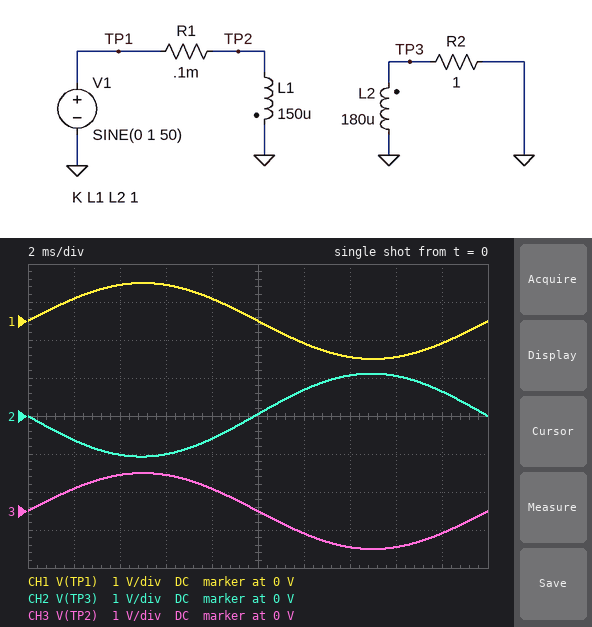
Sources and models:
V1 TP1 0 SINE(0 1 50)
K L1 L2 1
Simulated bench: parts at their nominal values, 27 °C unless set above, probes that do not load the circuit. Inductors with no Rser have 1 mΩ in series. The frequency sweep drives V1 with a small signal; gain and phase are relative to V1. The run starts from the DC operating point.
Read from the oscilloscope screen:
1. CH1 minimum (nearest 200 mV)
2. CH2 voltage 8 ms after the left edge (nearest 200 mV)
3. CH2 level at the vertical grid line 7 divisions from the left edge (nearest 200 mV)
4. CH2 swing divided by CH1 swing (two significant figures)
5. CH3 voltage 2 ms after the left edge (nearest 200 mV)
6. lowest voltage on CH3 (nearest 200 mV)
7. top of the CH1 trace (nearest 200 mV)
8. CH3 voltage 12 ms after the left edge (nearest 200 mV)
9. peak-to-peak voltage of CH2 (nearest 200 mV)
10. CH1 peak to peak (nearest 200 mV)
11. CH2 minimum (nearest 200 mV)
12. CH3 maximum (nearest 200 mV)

-1.0 V
-600 mV
1.0 V
1.1
600 mV
-1.0 V
1.0 V
-600 mV
2.2 V
2.0 V
-1.0 V
1.0 V
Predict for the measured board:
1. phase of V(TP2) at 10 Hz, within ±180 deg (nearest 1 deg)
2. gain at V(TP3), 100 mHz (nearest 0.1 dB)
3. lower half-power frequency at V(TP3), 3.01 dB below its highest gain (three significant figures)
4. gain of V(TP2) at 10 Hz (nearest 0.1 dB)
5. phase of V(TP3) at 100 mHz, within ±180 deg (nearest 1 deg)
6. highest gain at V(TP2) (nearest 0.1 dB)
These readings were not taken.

1 deg
-20.6 dB
1.17 Hz
0 dB
-95 deg
0 dB
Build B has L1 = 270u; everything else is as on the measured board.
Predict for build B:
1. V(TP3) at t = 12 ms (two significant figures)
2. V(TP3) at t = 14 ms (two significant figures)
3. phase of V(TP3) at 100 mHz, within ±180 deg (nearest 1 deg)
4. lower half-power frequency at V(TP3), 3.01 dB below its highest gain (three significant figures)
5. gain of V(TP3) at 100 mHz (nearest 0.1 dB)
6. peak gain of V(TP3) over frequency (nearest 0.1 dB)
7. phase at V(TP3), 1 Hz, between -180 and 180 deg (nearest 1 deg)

500 mV
790 mV
-99 deg
648 mHz
-18.1 dB
-1.8 dB
-147 deg
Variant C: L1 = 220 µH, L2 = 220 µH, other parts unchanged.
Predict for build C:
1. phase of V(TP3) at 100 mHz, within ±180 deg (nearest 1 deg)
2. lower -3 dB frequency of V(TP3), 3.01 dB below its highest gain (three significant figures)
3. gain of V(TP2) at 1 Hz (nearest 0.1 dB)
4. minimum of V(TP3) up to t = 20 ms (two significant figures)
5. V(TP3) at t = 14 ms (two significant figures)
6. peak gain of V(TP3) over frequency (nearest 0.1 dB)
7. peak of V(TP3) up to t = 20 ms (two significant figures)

-97 deg
795 mHz
-0.3 dB
-980 mV
970 mV
0 dB
1.0 V
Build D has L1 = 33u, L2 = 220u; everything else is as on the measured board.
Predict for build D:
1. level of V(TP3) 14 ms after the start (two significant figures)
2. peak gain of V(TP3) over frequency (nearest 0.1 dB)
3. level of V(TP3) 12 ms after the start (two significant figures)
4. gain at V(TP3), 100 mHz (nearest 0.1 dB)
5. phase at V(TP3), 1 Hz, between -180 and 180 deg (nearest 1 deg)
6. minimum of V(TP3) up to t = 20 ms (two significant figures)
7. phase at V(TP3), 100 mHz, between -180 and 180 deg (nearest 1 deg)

2.7 V
8.2 dB
1.9 V
-26.3 dB
-101 deg
-2.3 V
-91 deg
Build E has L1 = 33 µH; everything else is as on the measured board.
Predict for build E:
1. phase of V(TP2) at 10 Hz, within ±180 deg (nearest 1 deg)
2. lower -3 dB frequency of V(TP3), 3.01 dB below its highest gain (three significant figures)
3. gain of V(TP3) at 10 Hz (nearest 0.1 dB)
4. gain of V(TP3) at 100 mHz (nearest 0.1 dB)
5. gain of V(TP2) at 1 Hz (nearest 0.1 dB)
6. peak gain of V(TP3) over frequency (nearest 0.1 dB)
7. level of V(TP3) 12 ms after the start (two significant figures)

2 deg
5.27 Hz
6.2 dB
-27.1 dB
-0.8 dB
7.3 dB
1.7 V
